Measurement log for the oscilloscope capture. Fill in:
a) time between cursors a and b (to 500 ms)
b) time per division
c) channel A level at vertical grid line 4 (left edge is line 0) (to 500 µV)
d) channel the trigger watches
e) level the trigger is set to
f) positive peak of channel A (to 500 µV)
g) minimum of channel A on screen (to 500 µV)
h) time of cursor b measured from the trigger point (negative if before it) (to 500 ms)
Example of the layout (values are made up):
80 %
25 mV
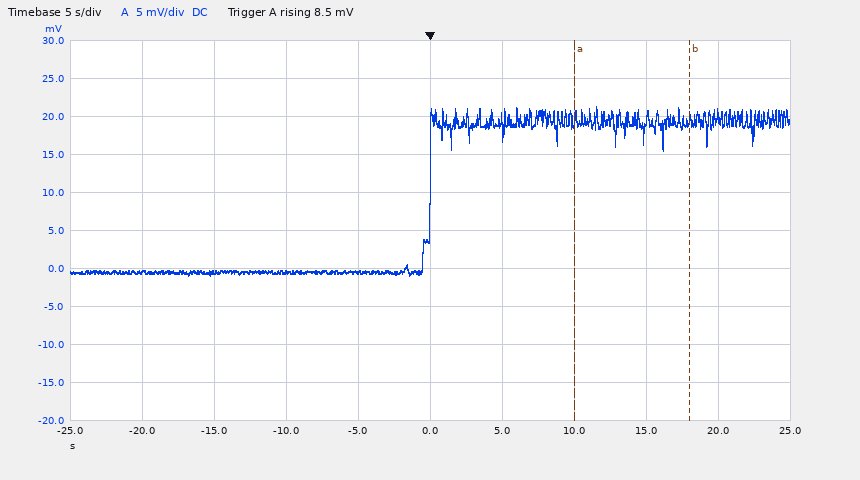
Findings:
8.0 s
5 s
-500 µV
channel A
8.5 mV
21.5 mV
-1.0 mV
+18.0 s
